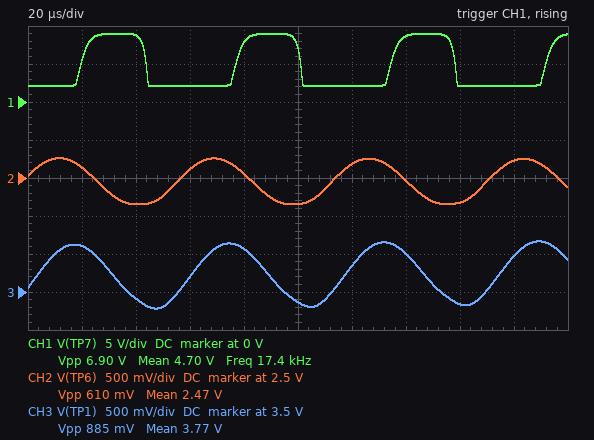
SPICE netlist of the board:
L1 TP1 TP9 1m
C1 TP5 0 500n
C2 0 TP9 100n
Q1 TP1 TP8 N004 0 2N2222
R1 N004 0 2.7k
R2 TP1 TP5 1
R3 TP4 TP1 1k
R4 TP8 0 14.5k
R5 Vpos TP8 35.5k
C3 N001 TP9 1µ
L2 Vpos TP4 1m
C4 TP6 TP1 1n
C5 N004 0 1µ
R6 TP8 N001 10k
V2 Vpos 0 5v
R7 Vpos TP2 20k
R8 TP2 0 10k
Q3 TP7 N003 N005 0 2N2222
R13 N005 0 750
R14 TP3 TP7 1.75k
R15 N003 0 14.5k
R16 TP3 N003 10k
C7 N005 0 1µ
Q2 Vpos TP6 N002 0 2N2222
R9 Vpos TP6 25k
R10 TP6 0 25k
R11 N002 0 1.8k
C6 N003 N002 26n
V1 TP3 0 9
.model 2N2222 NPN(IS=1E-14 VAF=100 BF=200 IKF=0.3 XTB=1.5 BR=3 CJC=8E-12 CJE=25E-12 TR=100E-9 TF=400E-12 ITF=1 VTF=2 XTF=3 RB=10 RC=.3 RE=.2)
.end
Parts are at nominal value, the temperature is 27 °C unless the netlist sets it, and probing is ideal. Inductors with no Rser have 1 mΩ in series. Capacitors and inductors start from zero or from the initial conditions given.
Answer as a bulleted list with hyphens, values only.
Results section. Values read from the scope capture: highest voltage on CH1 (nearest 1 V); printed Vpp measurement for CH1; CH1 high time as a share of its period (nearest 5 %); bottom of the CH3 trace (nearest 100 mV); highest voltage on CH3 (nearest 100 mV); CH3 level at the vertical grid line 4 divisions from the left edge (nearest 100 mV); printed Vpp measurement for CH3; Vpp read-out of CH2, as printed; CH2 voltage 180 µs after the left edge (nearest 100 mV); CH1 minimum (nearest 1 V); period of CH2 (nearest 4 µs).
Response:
- 9 V
- 6.90 V
- 40 %
- 3.3 V
- 4.2 V
- 4.1 V
- 885 mV
- 610 mV
- 2.7 V
- 2 V
- 56 µs
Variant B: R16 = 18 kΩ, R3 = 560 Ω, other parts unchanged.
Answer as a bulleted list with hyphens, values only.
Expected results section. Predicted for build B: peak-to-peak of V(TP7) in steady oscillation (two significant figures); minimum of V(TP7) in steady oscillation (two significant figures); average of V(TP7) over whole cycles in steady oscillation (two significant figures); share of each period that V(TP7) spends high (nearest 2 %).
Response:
- 7.5 V
- 1.5 V
- 5.6 V
- 56 %
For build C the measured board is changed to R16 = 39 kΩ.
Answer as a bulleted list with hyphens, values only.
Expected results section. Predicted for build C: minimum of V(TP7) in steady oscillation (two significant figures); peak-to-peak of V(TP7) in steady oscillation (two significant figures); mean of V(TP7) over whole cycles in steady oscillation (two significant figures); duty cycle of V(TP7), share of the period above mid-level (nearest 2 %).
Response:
- 1.0 V
- 8.0 V
- 6.8 V
- 74 %
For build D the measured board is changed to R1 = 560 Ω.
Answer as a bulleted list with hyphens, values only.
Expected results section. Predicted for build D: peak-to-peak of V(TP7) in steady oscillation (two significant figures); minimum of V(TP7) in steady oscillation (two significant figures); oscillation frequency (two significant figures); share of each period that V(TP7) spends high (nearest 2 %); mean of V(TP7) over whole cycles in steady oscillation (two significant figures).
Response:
- 7.1 V
- 1.9 V
- 17 kHz
- 52 %
- 5.5 V
